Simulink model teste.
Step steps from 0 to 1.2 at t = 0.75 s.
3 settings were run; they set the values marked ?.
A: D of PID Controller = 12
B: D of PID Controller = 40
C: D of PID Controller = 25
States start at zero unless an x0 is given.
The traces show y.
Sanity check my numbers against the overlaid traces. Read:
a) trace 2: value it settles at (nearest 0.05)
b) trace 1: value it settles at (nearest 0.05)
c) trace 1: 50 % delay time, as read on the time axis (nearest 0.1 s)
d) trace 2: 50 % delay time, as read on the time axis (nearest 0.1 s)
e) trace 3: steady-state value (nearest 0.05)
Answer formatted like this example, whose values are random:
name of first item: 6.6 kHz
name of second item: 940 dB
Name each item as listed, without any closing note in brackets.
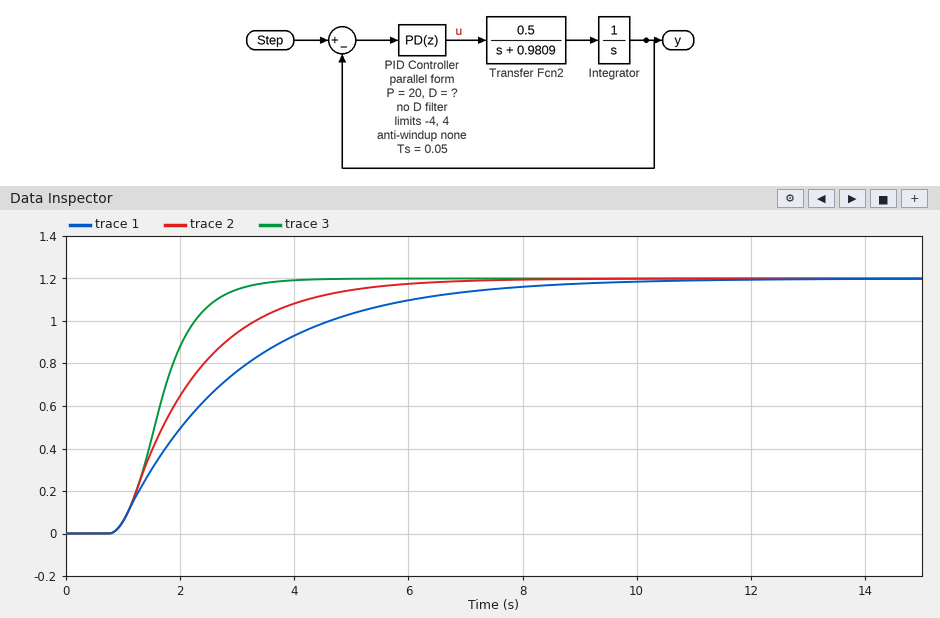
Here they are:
trace 2: value it settles at: 1.20
trace 1: value it settles at: 1.20
trace 1: 50 % delay time, as read on the time axis: 2.3 s
trace 2: 50 % delay time, as read on the time axis: 1.9 s
trace 3: steady-state value: 1.20
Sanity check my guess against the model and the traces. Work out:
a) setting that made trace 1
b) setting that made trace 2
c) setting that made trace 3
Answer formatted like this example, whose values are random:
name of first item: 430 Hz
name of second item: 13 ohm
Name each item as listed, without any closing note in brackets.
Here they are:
setting that made trace 1: B
setting that made trace 2: C
setting that made trace 3: A
